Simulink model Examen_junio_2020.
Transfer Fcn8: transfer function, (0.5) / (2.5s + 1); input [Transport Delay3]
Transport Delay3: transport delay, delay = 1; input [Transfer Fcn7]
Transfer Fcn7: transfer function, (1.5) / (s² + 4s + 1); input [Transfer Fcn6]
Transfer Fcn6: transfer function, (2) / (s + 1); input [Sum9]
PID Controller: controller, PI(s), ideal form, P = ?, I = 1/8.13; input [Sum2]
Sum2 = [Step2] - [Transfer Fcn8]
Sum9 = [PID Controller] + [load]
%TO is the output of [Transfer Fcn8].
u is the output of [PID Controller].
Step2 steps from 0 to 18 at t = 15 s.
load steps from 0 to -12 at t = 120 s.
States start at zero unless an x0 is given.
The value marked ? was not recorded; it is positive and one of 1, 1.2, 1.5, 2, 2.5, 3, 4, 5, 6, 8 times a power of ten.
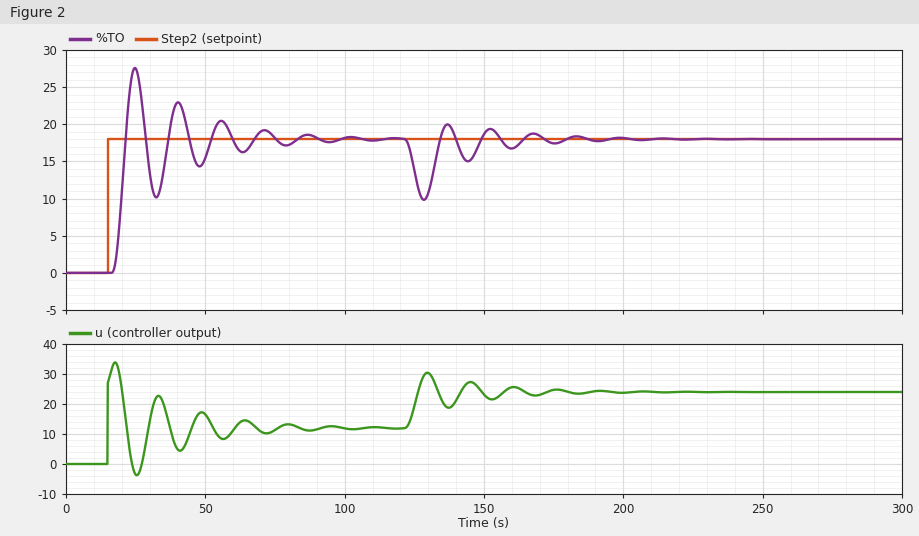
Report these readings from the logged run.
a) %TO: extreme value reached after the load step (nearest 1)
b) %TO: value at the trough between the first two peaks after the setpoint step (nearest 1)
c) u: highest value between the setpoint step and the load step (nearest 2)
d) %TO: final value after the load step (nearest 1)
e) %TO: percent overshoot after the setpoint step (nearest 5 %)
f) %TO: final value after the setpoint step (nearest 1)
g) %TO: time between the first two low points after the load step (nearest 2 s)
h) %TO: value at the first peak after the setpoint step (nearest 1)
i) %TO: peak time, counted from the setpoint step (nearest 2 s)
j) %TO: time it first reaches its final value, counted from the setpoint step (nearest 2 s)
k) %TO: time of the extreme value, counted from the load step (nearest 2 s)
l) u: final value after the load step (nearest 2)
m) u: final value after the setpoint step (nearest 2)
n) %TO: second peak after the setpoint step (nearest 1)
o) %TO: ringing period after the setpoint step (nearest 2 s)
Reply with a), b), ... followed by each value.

a) 10
b) 10
c) 34
d) 18
e) 55 %
f) 18
g) 16 s
h) 28
i) 10 s
j) 6 s
k) 8 s
l) 24
m) 12
n) 23
o) 16 s
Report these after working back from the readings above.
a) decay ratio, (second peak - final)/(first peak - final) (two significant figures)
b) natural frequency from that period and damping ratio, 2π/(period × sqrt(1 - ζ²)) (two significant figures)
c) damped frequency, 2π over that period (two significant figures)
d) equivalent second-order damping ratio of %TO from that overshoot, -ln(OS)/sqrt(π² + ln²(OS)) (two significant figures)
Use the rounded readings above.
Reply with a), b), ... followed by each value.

a) 0.50
b) 0.40 rad/s
c) 0.39 rad/s
d) 0.19
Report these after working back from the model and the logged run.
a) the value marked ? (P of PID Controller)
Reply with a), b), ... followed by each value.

a) 1.5
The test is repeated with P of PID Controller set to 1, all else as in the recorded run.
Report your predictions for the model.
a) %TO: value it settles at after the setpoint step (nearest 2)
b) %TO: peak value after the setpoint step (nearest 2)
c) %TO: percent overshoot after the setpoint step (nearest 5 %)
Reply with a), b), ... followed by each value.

a) 18
b) 22
c) 25 %
